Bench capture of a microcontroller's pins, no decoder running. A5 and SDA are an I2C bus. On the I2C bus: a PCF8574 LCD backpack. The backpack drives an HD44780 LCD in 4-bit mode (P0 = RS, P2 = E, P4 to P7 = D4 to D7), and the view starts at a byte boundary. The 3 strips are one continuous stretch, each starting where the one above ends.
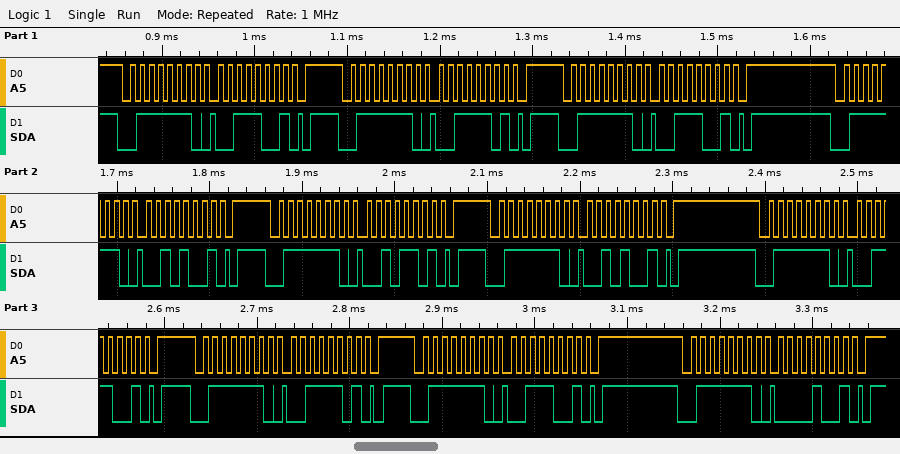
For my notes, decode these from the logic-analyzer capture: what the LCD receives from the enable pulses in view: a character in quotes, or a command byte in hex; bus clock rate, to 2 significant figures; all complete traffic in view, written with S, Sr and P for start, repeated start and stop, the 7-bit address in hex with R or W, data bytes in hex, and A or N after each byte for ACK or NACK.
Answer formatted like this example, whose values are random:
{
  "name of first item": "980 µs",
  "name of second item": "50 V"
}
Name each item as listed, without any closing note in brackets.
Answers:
{
  "what the LCD receives from the enable pulses in view: a character in quotes, or a command byte in hex": "'2'",
  "bus clock rate, to 2 significant figures": "100 kHz",
  "all complete traffic in view, written with S, Sr and P for start, repeated start and stop, the 7-bit address in hex with R or W, data bytes in hex, and A or N after each byte for ACK or NACK": "S 3FW A 39 A P S 3FW A 3D A P S 3FW A 39 A P S 3FW A 29 A P S 3FW A 2D A P S 3FW A 29 A P S 3FW A 39 A P S 3FW A 3D A P S 3FW A 39 A P S 3FW A 09 A P"
}
